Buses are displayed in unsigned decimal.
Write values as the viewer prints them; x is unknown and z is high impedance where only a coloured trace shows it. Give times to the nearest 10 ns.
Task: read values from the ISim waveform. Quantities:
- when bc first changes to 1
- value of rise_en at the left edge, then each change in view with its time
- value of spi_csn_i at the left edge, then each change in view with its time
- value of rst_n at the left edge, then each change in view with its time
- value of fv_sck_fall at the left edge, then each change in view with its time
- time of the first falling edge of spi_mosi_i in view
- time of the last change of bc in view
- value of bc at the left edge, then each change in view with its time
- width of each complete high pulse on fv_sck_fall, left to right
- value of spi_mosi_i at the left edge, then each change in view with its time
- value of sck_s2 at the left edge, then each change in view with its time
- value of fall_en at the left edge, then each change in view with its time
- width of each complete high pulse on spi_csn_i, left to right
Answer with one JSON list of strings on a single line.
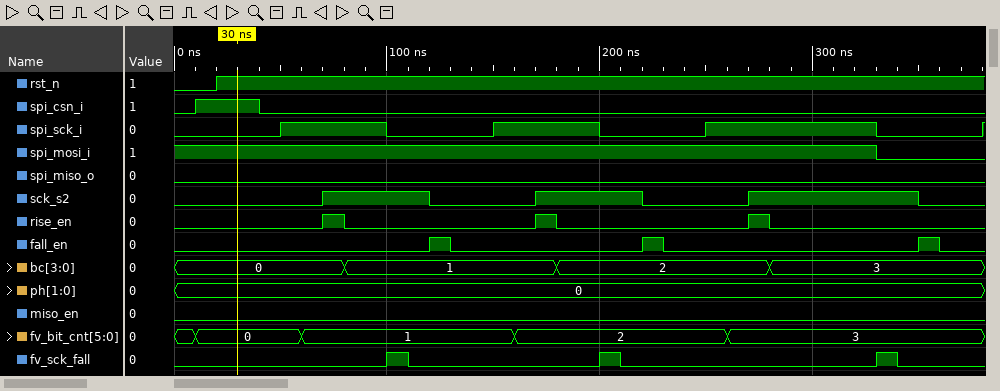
["80 ns", "0, 1 at 70 ns, 0 at 80 ns, 1 at 170 ns, 0 at 180 ns, 1 at 270 ns, 0 at 280 ns", "0, 1 at 10 ns, 0 at 40 ns", "0, 1 at 20 ns", "0, 1 at 100 ns, 0 at 110 ns, 1 at 200 ns, 0 at 210 ns, 1 at 330 ns, 0 at 340 ns", "330 ns", "280 ns", "0, 1 at 80 ns, 2 at 180 ns, 3 at 280 ns", "10 ns, 10 ns, 10 ns", "1, 0 at 330 ns", "0, 1 at 70 ns, 0 at 120 ns, 1 at 170 ns, 0 at 220 ns, 1 at 270 ns, 0 at 350 ns", "0, 1 at 120 ns, 0 at 130 ns, 1 at 220 ns, 0 at 230 ns, 1 at 350 ns, 0 at 360 ns", "30 ns"]
